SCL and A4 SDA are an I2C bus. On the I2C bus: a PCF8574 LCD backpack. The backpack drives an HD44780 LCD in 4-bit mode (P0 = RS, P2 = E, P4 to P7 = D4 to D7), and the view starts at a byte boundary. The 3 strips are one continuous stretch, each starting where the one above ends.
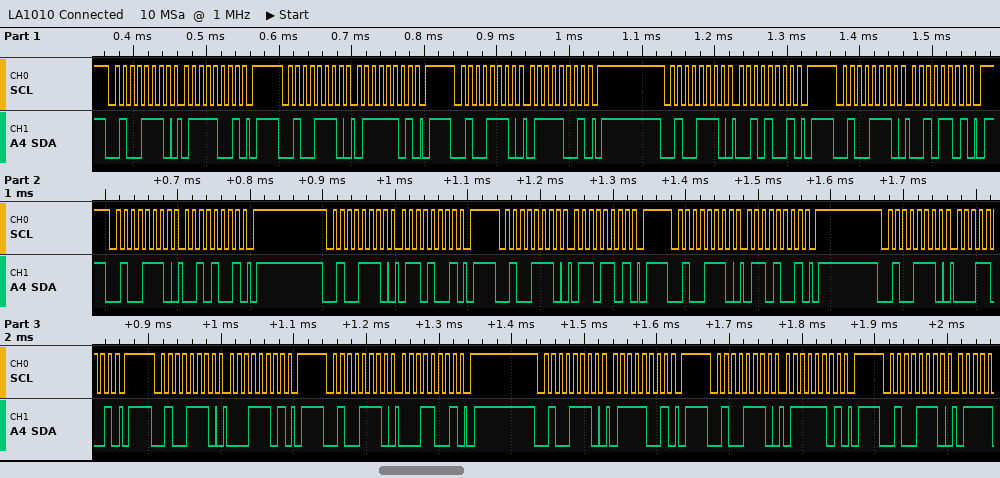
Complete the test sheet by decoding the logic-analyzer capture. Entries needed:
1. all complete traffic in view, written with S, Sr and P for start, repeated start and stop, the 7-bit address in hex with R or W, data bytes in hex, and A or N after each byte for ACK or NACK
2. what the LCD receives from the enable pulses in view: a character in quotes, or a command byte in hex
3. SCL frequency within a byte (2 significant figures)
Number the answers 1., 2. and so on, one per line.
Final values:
1. S 27W A 79 A P S 27W A 7D A P S 27W A 79 A P S 27W A 29 A P S 27W A 2D A P S 27W A 29 A P S 27W A 69 A P S 27W A 6D A P S 27W A 69 A P S 27W A 19 A P S 27W A 1D A P S 27W A 19 A P S 27W A 79 A P S 27W A 7D A P S 27W A
2. 'r' 'a'
3. 100 kHz
